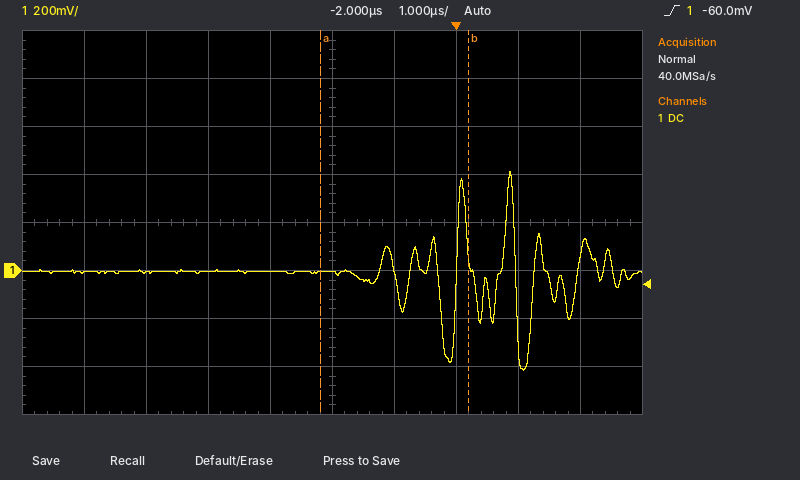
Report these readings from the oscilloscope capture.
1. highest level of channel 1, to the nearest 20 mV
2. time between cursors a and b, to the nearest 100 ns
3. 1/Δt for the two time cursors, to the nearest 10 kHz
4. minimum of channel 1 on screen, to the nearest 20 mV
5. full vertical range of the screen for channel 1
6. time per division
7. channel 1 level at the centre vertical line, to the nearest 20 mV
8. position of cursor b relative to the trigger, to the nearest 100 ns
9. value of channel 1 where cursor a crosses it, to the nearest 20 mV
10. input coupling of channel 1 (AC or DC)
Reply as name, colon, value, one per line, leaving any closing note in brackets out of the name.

highest level of channel 1, to the nearest 20 mV: 420 mV
time between cursors a and b, to the nearest 100 ns: 2.4 µs
1/Δt for the two time cursors, to the nearest 10 kHz: 420 kHz
minimum of channel 1 on screen, to the nearest 20 mV: -420 mV
full vertical range of the screen for channel 1: 1.6 V
time per division: 1 µs
channel 1 level at the centre vertical line, to the nearest 20 mV: 0 mV
position of cursor b relative to the trigger, to the nearest 100 ns: +200 ns
value of channel 1 where cursor a crosses it, to the nearest 20 mV: 0 mV
input coupling of channel 1: DC
